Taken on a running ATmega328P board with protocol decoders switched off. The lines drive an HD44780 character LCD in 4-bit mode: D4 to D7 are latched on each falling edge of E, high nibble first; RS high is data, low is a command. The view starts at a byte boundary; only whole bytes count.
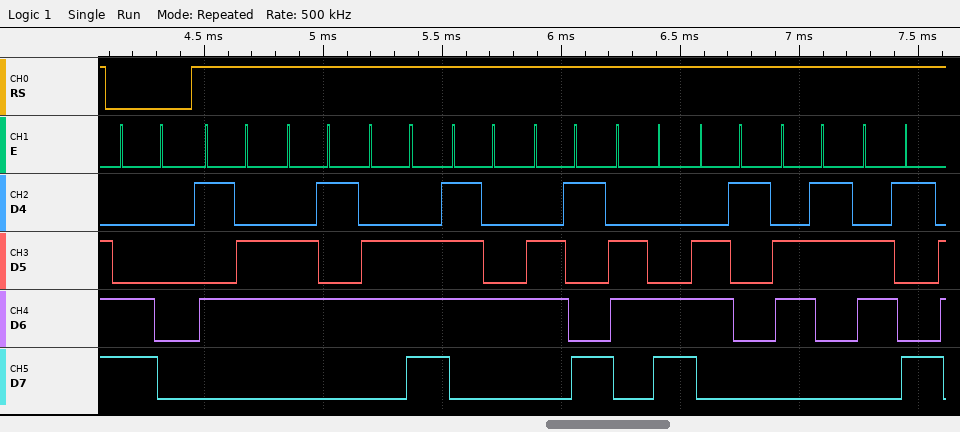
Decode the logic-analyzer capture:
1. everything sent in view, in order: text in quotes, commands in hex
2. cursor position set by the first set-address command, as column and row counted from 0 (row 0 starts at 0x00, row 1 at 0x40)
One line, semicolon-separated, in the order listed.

0xC0 "Ventilaci"; column 0, row 1
